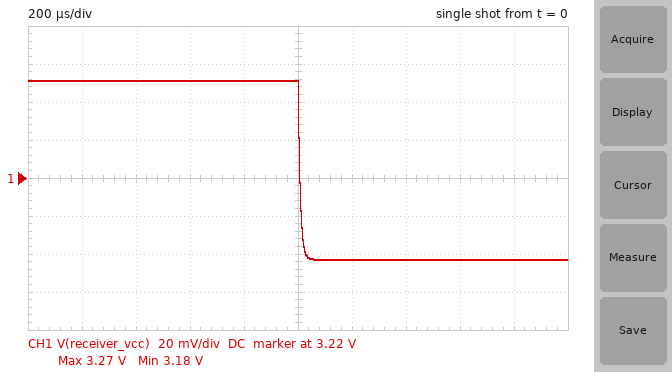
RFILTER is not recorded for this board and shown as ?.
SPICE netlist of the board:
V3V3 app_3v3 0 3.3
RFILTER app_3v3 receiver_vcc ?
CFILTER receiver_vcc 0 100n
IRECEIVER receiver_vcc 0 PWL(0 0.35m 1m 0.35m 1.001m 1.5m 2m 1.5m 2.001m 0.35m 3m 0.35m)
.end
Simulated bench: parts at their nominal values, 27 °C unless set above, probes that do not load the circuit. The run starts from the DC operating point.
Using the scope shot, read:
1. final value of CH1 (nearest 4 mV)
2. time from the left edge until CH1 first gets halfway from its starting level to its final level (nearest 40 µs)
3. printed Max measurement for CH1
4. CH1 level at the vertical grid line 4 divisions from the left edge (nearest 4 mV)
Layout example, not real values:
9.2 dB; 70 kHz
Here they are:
3.176 V; 1.00 ms; 3.27 V; 3.272 V
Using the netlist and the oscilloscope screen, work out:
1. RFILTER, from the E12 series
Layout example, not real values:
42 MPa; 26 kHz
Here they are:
82 Ω
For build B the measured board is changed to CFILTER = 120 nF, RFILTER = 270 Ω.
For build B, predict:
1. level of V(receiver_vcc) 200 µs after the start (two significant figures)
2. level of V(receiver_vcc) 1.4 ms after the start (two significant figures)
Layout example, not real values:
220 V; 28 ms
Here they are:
3.2 V; 2.9 V
